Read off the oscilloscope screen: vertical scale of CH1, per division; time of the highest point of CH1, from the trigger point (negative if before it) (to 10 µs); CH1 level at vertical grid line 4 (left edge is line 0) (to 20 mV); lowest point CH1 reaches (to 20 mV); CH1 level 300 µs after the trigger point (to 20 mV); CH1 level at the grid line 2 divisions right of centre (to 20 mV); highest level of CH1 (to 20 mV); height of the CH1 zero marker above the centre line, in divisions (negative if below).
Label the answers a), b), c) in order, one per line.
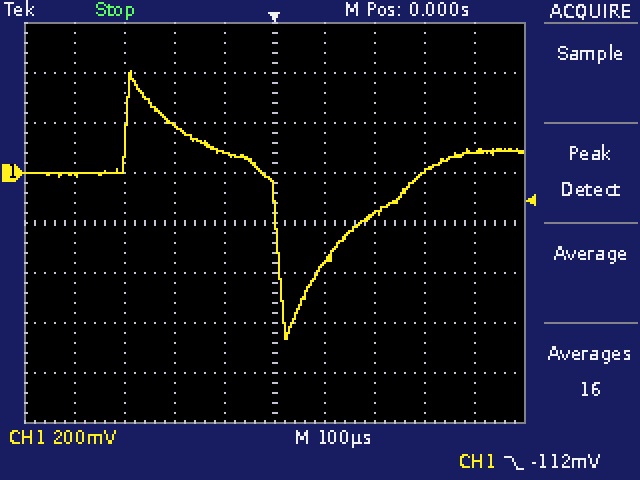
a) 200 mV
b) -290 µs
c) 80 mV
d) -660 mV
e) 0 mV
f) -160 mV
g) 400 mV
h) +1.0 div
